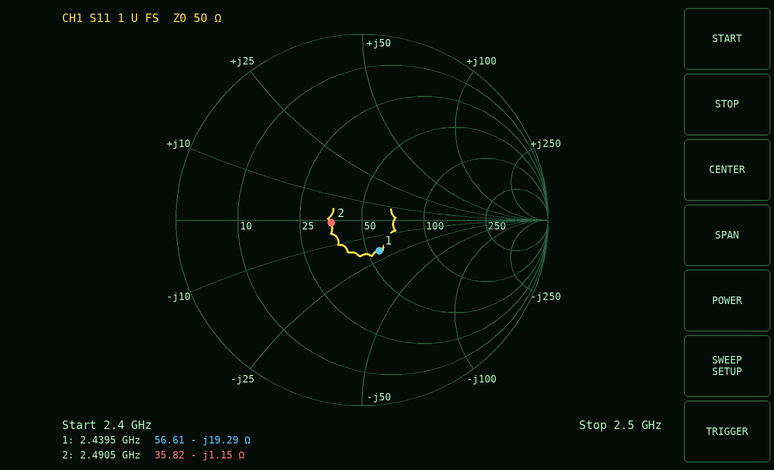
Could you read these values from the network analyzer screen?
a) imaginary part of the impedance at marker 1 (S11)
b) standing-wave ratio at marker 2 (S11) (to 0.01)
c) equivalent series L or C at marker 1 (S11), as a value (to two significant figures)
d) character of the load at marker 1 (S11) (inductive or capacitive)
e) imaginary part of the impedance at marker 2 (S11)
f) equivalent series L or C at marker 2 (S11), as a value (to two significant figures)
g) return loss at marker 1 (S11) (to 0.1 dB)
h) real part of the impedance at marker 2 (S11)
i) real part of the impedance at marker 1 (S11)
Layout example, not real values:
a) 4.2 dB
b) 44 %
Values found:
a) -19.29 Ω
b) 1.40
c) 3.4 pF
d) capacitive
e) -1.15 Ω
f) 56 pF
g) 14.5 dB
h) 35.82 Ω
i) 56.61 Ω
